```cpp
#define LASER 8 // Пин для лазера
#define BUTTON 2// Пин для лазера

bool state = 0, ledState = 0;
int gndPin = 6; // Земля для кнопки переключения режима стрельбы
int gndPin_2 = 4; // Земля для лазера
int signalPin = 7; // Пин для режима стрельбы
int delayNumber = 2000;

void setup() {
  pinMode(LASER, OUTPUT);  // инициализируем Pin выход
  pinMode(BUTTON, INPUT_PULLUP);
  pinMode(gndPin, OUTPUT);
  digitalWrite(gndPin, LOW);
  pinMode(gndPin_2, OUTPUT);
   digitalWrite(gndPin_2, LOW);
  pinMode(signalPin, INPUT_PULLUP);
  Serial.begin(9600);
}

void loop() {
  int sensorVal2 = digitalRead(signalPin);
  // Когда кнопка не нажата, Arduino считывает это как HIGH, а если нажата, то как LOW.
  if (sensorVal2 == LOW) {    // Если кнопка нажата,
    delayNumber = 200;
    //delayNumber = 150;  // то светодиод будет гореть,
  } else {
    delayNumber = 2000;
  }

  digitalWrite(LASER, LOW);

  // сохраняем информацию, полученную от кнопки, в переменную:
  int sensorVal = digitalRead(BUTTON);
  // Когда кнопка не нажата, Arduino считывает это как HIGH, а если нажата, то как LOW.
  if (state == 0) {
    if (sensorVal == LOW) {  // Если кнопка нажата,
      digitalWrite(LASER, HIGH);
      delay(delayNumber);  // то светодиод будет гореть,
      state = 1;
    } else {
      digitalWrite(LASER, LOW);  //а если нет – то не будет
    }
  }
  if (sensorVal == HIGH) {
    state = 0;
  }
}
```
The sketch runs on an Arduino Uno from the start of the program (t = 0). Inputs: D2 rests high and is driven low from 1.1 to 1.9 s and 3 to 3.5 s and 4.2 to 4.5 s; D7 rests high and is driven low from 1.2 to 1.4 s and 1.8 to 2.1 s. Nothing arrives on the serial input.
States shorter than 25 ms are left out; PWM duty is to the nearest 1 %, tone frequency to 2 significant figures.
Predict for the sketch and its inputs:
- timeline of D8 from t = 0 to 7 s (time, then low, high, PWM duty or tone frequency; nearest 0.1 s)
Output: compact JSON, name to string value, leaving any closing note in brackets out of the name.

{"timeline of D8 from t = 0 to 7 s": "0 s low; 1.1 s high; 3.1 s low; 4.2 s high; 6.2 s low"}
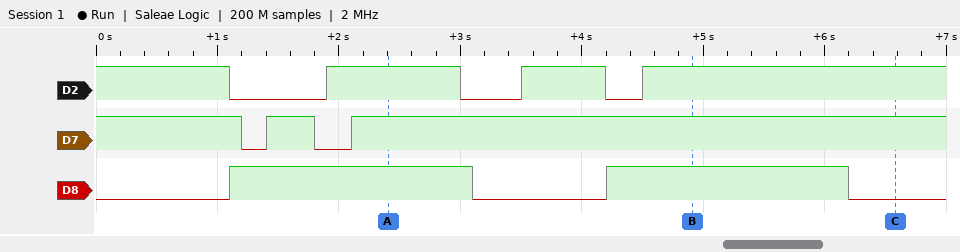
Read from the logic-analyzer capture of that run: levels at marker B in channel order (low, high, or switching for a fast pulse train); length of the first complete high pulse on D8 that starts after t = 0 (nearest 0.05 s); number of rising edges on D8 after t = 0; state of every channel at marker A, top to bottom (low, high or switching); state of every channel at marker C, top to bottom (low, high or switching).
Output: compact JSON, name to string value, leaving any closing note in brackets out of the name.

{"levels at marker B in channel order": "D2 high, D7 high, D8 high", "length of the first complete high pulse on D8 that starts after t = 0": "2.00 s", "number of rising edges on D8 after t = 0": "2", "state of every channel at marker A, top to bottom": "D2 high, D7 high, D8 high", "state of every channel at marker C, top to bottom": "D2 high, D7 high, D8 low"}
